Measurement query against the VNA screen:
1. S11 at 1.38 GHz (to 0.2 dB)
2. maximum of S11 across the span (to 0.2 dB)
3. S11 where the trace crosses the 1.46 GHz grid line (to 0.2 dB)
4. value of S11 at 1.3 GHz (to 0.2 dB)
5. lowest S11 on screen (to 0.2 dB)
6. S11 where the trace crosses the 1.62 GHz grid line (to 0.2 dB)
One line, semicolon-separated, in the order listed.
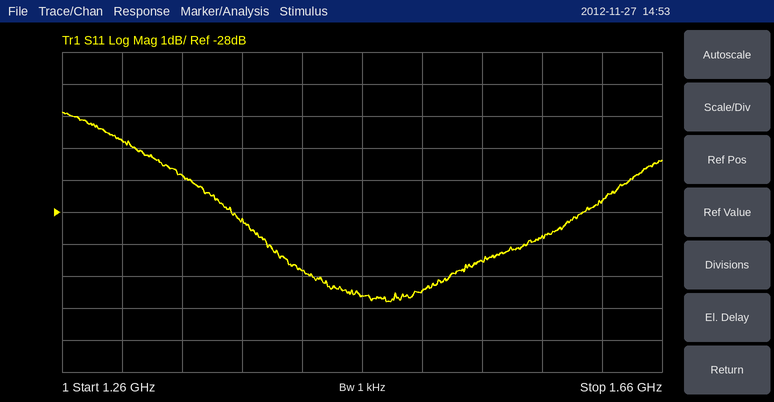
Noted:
-28.2 dB; -24.8 dB; -30.6 dB; -25.8 dB; -30.8 dB; -27.6 dB
